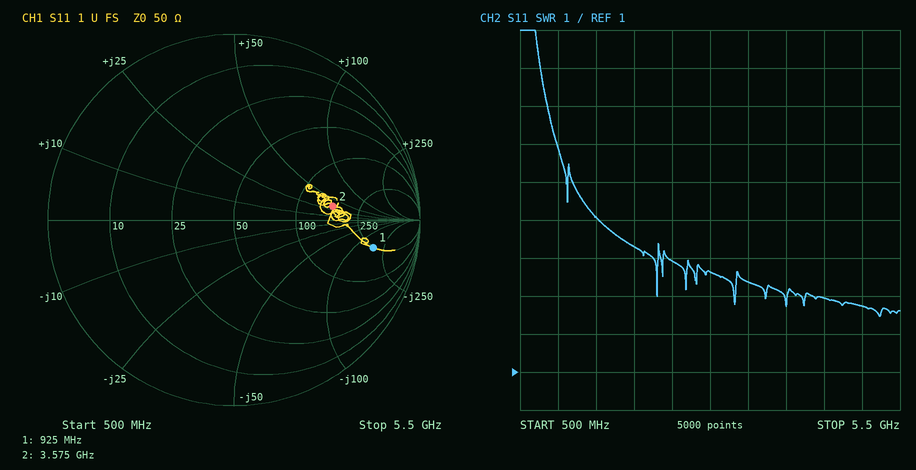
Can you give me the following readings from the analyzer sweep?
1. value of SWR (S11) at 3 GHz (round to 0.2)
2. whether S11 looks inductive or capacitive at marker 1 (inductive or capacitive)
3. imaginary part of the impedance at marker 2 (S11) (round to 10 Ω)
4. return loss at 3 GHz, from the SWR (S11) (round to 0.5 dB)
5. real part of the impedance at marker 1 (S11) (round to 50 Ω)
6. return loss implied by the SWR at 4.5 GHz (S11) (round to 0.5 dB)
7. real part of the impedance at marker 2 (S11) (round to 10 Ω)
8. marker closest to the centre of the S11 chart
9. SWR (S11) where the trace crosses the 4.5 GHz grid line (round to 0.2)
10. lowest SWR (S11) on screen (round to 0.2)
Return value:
3.6
capacitive
+30 Ω
5.0 dB
250 Ω
6.0 dB
160 Ω
marker 2
3.0
2.4
